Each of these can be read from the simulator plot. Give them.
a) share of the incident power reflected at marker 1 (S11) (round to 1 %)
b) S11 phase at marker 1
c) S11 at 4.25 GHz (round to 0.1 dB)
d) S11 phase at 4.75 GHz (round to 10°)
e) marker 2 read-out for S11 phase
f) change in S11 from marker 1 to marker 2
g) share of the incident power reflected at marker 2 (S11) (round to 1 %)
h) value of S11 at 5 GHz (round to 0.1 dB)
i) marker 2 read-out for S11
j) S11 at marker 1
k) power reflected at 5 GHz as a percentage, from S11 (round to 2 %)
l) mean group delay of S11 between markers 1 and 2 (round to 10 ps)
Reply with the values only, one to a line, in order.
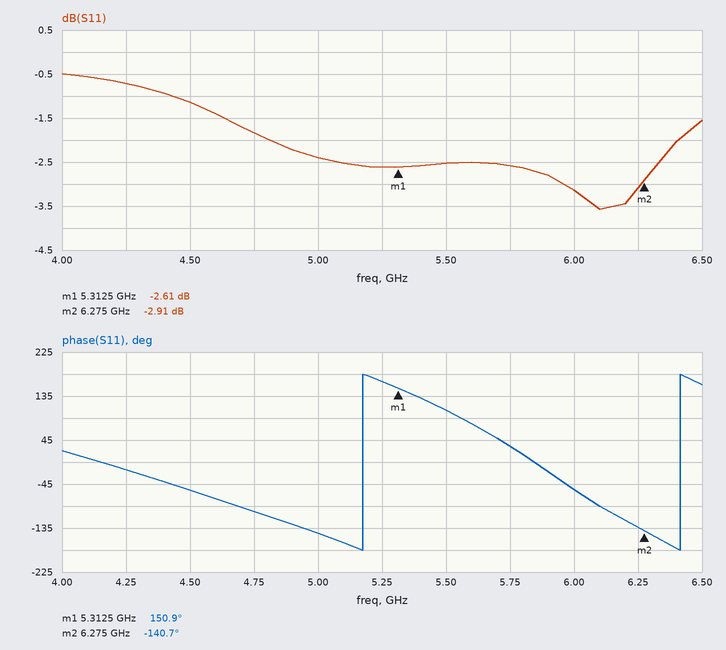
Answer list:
55 %
150.9°
-0.7 dB
-100°
-140.7°
-0.30 dB
51 %
-2.4 dB
-2.91 dB
-2.61 dB
58 %
840 ps
